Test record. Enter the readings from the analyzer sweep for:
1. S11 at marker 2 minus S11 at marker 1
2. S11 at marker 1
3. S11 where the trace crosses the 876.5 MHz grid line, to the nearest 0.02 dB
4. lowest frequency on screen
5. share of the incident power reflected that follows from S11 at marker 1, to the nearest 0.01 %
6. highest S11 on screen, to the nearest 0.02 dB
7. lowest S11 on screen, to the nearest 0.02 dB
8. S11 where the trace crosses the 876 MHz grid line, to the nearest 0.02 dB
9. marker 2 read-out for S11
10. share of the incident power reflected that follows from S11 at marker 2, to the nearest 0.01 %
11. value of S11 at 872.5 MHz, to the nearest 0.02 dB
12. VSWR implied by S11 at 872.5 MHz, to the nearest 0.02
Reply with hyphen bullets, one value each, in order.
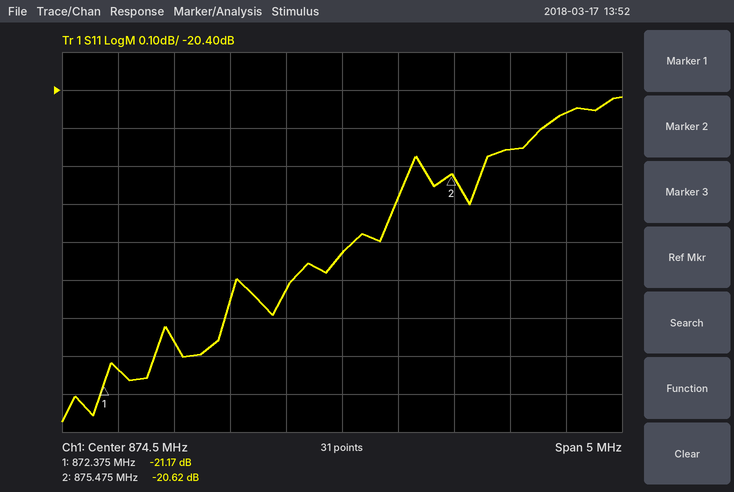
- 0.55 dB
- -21.17 dB
- -20.46 dB
- 872 MHz
- 0.76 %
- -20.42 dB
- -21.28 dB
- -20.56 dB
- -20.62 dB
- 0.87 %
- -21.14 dB
- 1.20
